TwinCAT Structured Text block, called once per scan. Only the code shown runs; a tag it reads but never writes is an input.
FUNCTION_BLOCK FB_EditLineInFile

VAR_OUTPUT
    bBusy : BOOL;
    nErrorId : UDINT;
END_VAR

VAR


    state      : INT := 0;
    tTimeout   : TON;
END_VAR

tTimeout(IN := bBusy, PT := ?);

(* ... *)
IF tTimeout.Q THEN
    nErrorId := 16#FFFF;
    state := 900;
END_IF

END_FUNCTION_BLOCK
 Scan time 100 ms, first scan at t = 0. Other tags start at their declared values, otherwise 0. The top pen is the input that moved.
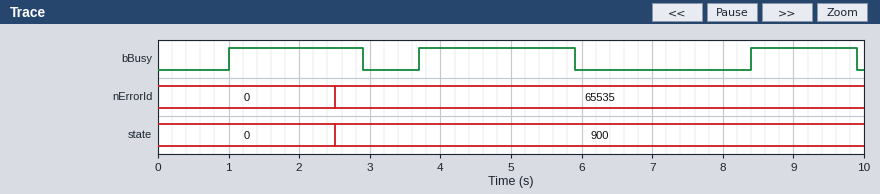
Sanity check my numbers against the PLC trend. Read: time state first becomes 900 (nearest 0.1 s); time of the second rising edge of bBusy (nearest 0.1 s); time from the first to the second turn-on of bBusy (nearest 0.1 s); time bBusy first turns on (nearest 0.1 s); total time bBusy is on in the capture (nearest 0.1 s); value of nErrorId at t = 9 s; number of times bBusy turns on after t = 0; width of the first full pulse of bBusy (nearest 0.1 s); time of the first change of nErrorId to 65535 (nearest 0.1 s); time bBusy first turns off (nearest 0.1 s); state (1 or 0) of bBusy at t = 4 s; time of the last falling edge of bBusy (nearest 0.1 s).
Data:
2.5 s
3.7 s
2.7 s
1.0 s
5.6 s
65535
3
1.9 s
2.5 s
2.9 s
1
9.9 s
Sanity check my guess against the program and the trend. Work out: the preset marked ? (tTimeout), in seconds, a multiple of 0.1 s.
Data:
1.5 s
